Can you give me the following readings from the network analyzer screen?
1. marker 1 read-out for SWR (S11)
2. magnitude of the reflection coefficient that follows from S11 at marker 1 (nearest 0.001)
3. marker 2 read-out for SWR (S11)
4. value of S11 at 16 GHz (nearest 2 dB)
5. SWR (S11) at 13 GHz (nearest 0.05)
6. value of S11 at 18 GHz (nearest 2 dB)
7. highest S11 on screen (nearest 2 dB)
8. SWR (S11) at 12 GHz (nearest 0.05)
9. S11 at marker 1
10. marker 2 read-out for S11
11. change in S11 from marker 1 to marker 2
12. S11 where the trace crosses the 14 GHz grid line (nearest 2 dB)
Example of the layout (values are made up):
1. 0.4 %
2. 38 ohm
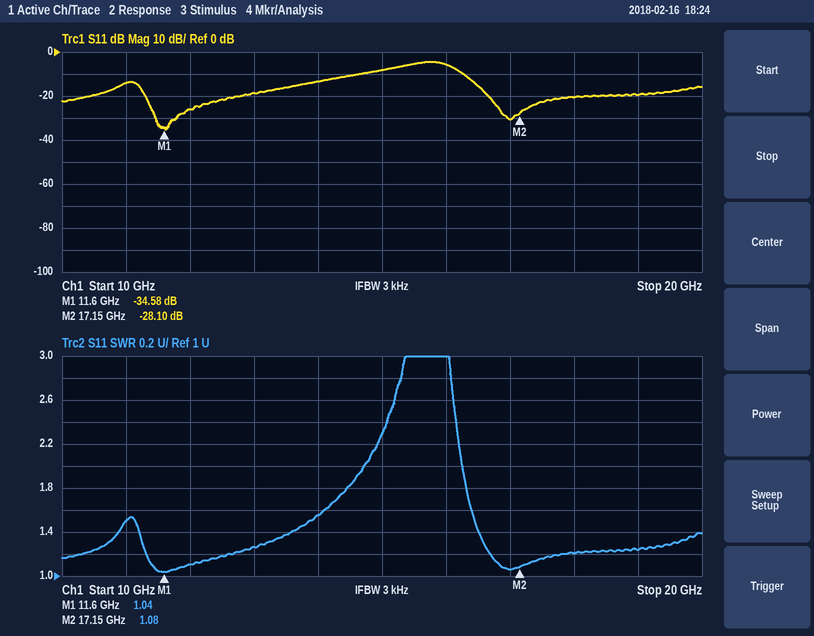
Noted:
1. 1.04
2. 0.019
3. 1.08
4. -6 dB
5. 1.25
6. -20 dB
7. -4 dB
8. 1.10
9. -34.58 dB
10. -28.10 dB
11. 6.48 dB
12. -14 dB
